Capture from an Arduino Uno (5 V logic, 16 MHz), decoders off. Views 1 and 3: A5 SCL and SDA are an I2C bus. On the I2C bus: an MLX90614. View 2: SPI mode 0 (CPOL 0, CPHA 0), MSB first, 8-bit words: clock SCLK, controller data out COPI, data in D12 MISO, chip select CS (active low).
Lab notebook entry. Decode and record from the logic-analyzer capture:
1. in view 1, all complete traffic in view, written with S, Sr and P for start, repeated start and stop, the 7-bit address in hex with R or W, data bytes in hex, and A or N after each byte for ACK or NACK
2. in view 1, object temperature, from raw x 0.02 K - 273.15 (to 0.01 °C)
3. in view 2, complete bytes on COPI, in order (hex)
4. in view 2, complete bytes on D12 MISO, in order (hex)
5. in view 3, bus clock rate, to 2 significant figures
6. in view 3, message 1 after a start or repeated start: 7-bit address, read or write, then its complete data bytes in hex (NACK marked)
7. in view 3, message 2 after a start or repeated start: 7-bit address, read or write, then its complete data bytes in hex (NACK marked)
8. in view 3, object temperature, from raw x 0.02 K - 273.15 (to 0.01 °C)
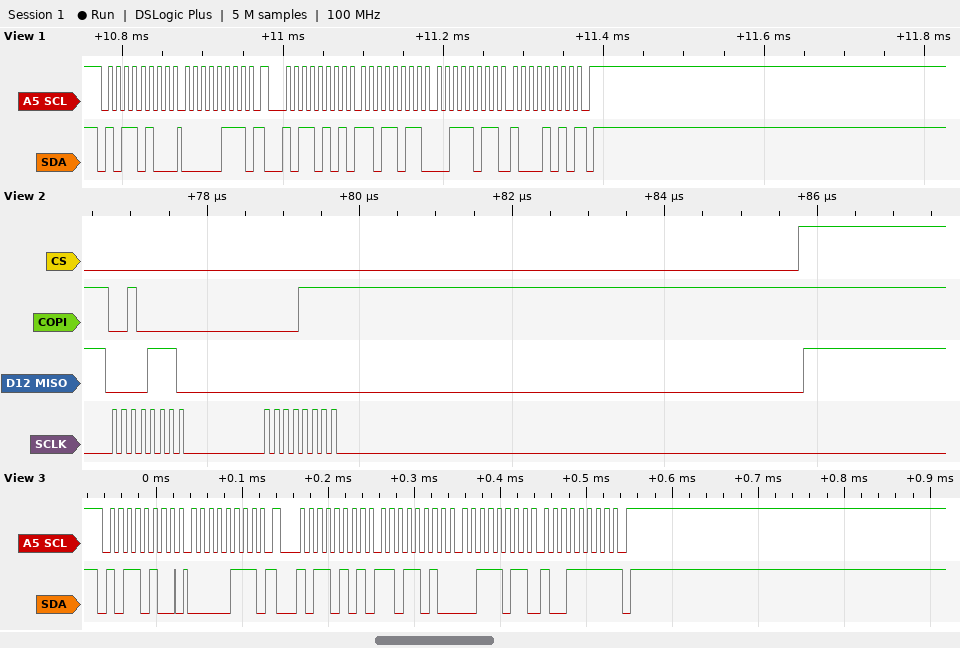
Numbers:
S 5AW A 07 A Sr 5AR A DB A 3B A 8A N P
33.31 °C
20 0F
0E 00
100 kHz
0x5A write: 07
0x5A read: DA 3B 9F NACK
33.29 °C
